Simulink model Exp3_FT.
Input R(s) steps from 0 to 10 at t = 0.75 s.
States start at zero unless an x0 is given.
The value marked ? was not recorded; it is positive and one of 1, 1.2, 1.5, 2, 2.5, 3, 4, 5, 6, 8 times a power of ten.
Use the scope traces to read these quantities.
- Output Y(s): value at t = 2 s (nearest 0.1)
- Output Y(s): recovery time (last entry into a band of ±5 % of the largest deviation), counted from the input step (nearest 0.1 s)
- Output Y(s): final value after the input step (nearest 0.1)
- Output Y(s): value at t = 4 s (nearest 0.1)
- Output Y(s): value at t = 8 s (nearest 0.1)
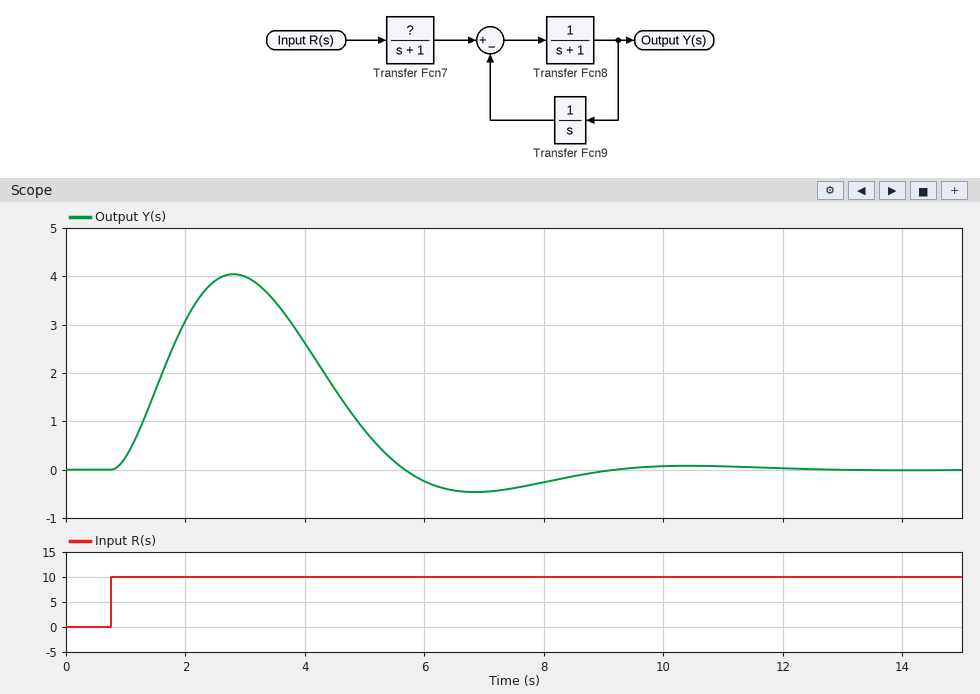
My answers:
3.1
7.5 s
0.0
2.6
-0.3
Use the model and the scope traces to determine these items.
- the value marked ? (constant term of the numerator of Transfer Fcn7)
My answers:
1
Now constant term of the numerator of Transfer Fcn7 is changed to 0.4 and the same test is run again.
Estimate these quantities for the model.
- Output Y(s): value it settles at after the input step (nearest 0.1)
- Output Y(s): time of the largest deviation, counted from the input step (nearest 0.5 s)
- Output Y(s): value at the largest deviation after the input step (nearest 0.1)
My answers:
0.0
2.0 s
1.6
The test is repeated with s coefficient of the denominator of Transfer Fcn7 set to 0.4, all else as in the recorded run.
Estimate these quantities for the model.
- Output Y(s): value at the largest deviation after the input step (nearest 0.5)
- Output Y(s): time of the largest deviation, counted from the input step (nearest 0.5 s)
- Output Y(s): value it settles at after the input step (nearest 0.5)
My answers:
5.0
1.5 s
0.0
